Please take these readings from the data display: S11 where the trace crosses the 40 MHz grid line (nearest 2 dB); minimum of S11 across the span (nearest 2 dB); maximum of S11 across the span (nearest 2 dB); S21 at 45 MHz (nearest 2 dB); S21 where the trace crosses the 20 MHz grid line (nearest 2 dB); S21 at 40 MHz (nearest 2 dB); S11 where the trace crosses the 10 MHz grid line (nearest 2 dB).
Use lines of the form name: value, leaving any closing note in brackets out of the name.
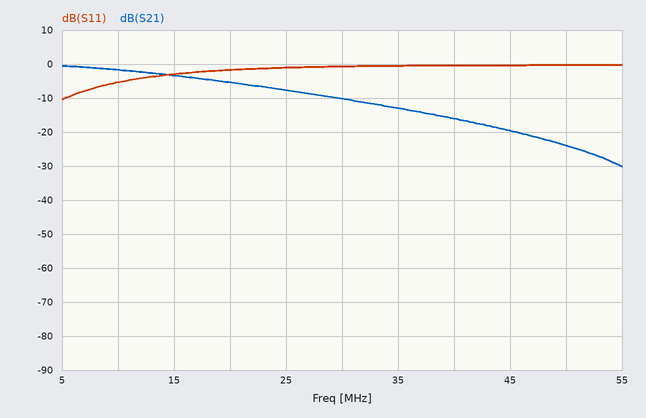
S11 where the trace crosses the 40 MHz grid line: 0 dB
minimum of S11 across the span: -10 dB
maximum of S11 across the span: 0 dB
S21 at 45 MHz: -20 dB
S21 where the trace crosses the 20 MHz grid line: -6 dB
S21 at 40 MHz: -16 dB
S11 where the trace crosses the 10 MHz grid line: -6 dB
